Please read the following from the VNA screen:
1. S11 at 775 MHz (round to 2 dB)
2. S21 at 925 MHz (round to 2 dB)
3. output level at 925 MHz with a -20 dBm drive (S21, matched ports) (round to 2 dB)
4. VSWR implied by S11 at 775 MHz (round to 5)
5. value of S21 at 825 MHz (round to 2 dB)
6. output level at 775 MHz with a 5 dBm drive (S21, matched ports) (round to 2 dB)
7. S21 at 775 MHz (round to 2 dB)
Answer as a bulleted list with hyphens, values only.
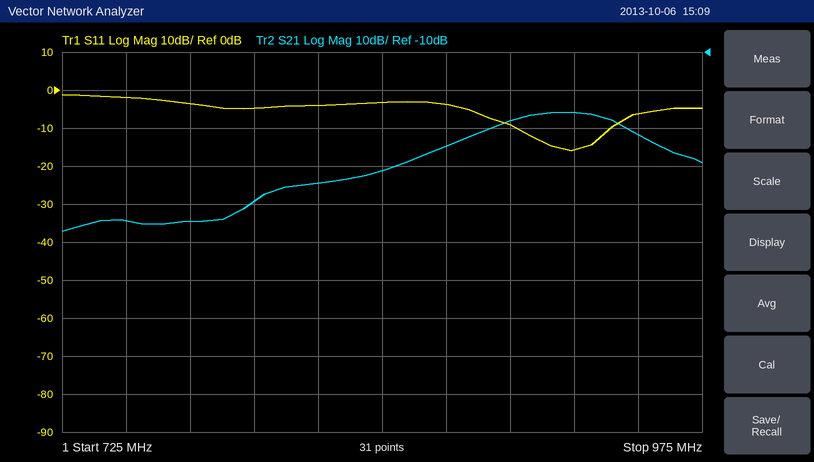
- -4 dB
- -26 dB
- -46 dBm
- 5
- -44 dB
- -50 dBm
- -54 dB
